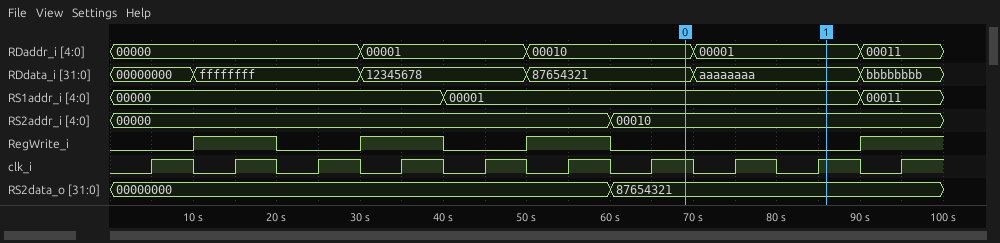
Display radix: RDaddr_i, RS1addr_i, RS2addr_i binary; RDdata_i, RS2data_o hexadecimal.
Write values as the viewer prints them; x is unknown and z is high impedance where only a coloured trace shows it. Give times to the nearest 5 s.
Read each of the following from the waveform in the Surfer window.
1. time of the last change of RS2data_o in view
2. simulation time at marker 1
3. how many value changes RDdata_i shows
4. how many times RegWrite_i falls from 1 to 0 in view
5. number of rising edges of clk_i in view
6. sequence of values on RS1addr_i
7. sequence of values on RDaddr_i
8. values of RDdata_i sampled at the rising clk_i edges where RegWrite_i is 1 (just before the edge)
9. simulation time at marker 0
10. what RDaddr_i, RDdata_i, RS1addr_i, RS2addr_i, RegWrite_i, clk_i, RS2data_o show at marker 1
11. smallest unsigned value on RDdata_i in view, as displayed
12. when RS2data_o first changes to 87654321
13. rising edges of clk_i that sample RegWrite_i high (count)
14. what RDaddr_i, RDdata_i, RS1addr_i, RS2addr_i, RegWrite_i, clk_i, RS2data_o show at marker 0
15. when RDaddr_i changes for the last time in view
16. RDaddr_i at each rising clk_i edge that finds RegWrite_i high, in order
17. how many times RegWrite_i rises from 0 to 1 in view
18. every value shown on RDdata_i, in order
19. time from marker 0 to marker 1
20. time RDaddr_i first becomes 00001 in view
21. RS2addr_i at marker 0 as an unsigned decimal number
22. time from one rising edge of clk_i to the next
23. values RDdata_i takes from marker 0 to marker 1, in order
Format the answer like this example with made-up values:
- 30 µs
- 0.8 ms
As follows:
- 60 s
- 85 s
- 5
- 3
- 10
- 00000, 00001, 00011
- 00000, 00001, 00010, 00001, 00011
- ffffffff, 12345678, 87654321, bbbbbbbb
- 70 s
- RDaddr_i=00001, RDdata_i=aaaaaaaa, RS1addr_i=00001, RS2addr_i=00010, RegWrite_i=0, clk_i=1, RS2data_o=87654321
- 00000000
- 60 s
- 4
- RDaddr_i=00010, RDdata_i=87654321, RS1addr_i=00001, RS2addr_i=00010, RegWrite_i=0, clk_i=1, RS2data_o=87654321
- 90 s
- 00000, 00001, 00010, 00011
- 4
- 00000000, ffffffff, 12345678, 87654321, aaaaaaaa, bbbbbbbb
- 15 s
- 30 s
- 2
- 10 s
- 87654321, aaaaaaaa
